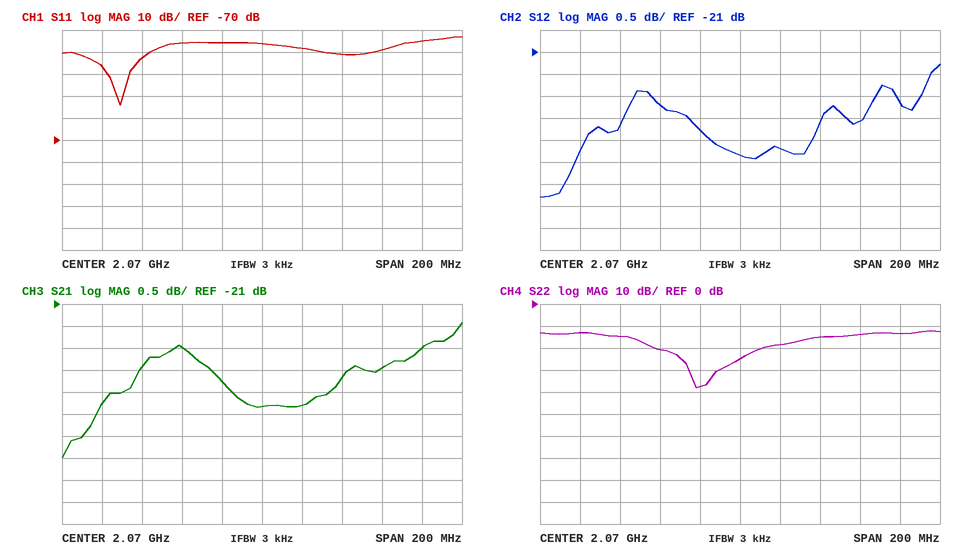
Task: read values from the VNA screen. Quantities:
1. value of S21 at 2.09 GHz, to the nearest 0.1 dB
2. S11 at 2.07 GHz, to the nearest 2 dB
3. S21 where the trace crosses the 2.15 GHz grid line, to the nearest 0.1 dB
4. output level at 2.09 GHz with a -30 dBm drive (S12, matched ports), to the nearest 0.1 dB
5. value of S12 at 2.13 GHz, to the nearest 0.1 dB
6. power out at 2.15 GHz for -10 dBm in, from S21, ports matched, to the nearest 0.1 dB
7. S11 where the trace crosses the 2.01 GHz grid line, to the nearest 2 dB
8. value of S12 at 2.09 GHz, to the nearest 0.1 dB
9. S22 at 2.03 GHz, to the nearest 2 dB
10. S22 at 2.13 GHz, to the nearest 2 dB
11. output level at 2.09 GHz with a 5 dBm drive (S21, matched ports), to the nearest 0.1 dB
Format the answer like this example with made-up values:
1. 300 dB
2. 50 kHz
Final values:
1. -23.3 dB
2. -26 dB
3. -22.0 dB
4. -53.2 dBm
5. -22.6 dB
6. -32.0 dBm
7. -32 dB
8. -23.2 dB
9. -20 dB
10. -14 dB
11. -18.3 dBm
